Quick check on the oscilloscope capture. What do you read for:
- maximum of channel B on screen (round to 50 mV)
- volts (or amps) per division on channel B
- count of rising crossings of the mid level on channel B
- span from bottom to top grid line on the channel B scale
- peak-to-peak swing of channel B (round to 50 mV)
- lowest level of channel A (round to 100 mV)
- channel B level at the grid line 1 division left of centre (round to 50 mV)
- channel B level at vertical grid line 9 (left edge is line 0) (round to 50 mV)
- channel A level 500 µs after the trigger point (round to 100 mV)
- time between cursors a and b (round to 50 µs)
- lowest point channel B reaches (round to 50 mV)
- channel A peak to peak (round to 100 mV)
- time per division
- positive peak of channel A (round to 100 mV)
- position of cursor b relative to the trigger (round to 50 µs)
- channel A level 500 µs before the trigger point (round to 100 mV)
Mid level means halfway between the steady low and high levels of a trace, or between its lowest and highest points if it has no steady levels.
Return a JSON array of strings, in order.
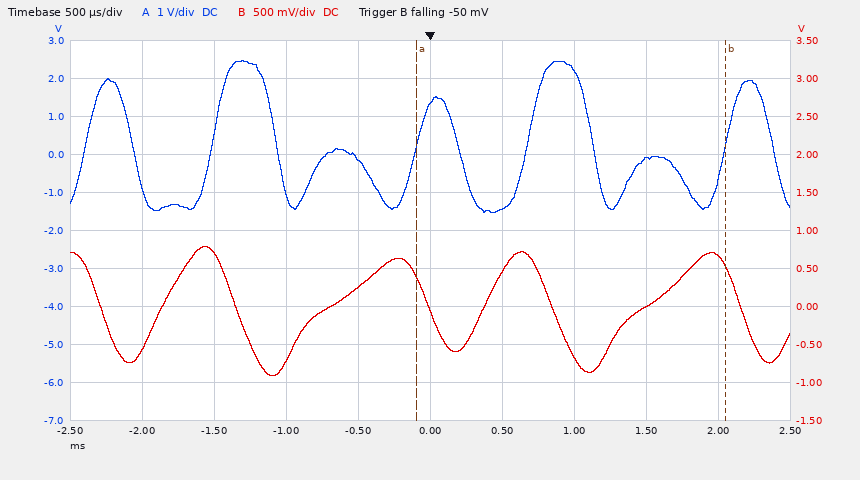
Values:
["800 mV", "500 mV", "4", "5 V", "1.70 V", "-1.5 V", "250 mV", "650 mV", "-1.4 V", "2.15 ms", "-900 mV", "4.0 V", "500 µs", "2.5 V", "+2.05 ms", "-100 mV"]
